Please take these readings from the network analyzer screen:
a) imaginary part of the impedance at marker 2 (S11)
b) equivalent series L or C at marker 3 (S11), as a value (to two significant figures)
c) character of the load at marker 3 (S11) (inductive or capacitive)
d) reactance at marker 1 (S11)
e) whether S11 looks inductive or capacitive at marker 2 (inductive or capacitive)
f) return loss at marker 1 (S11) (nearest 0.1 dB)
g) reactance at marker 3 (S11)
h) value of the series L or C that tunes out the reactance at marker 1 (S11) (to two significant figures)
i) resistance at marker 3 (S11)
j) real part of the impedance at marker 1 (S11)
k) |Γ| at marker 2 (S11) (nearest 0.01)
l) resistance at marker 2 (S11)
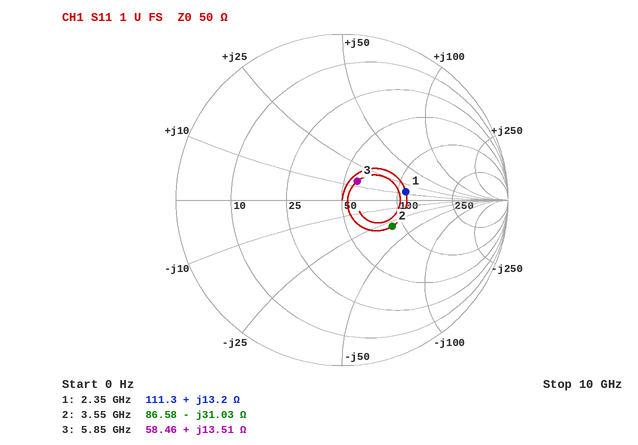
-31.03 Ω
370 pH
inductive
+13.2 Ω
capacitive
8.2 dB
+13.51 Ω
5.1 pF
58.46 Ω
111.3 Ω
0.34
86.58 Ω
